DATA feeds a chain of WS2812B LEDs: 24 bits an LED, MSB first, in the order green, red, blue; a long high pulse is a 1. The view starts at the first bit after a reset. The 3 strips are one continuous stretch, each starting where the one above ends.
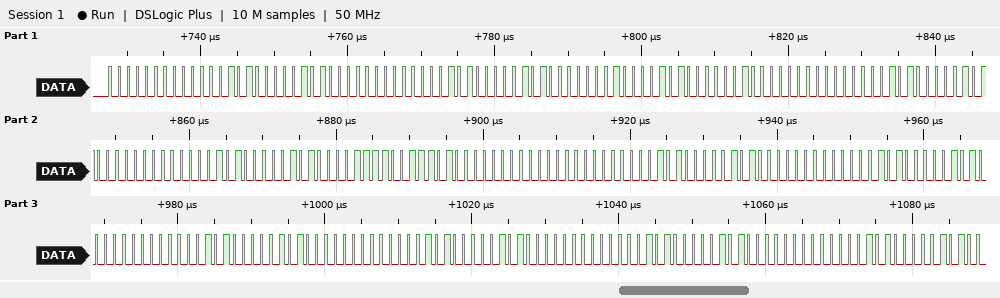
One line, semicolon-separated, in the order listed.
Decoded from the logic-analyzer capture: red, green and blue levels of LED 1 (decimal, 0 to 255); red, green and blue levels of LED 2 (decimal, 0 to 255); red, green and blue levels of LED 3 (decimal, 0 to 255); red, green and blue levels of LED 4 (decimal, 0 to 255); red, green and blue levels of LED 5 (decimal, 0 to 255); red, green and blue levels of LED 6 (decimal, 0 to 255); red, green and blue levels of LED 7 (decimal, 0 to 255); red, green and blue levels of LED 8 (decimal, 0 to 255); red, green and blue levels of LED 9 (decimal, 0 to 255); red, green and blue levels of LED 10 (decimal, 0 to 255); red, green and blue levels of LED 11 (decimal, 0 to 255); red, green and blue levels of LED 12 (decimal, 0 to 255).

5, 0, 5; 5, 0, 5; 10, 1, 4; 5, 0, 5; 5, 0, 5; 58, 15, 0; 5, 0, 5; 5, 0, 5; 5, 0, 5; 5, 0, 5; 5, 0, 5; 5, 0, 5
